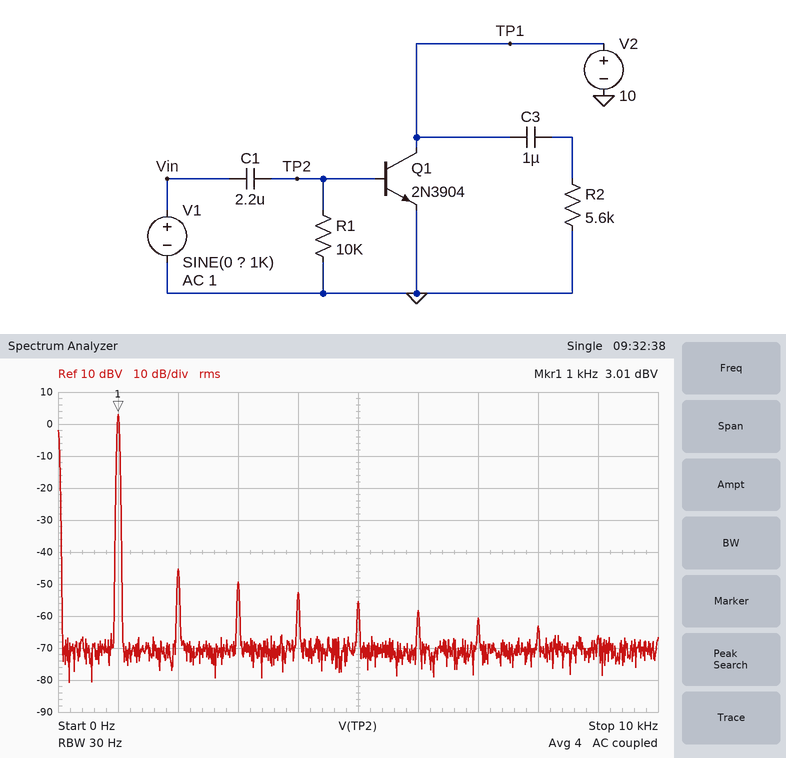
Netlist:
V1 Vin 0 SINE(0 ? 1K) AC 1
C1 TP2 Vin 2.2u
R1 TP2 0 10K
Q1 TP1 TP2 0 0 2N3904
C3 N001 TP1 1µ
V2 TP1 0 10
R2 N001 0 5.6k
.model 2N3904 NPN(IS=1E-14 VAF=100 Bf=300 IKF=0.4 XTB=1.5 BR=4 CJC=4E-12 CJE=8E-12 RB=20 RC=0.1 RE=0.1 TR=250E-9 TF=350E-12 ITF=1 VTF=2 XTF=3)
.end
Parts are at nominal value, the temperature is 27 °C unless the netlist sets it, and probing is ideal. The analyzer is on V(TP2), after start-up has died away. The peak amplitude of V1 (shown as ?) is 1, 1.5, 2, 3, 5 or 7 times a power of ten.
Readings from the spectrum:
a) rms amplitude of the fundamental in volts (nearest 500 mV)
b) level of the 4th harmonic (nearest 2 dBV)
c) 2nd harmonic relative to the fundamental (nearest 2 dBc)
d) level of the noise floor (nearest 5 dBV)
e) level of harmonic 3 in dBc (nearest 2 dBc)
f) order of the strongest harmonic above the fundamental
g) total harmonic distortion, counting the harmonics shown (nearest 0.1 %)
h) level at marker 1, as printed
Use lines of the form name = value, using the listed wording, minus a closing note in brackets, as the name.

rms amplitude of the fundamental in volts = 1.5 V
level of the 4th harmonic = -52 dBV
2nd harmonic relative to the fundamental = -48 dBc
level of the noise floor = -70 dBV
level of harmonic 3 in dBc = -52 dBc
order of the strongest harmonic above the fundamental = 2
total harmonic distortion, counting the harmonics shown = 0.5 %
level at marker 1, as printed = 3.01 dBV
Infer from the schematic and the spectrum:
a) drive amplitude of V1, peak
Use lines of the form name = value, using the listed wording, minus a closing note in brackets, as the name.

drive amplitude of V1, peak = 2 V
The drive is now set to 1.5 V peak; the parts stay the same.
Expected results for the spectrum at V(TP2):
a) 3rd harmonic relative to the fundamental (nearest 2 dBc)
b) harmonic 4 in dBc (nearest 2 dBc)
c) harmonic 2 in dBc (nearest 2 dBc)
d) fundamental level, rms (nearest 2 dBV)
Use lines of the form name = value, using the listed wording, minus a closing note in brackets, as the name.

3rd harmonic relative to the fundamental = -54 dBc
harmonic 4 in dBc = -58 dBc
harmonic 2 in dBc = -50 dBc
fundamental level, rms = 0 dBV
